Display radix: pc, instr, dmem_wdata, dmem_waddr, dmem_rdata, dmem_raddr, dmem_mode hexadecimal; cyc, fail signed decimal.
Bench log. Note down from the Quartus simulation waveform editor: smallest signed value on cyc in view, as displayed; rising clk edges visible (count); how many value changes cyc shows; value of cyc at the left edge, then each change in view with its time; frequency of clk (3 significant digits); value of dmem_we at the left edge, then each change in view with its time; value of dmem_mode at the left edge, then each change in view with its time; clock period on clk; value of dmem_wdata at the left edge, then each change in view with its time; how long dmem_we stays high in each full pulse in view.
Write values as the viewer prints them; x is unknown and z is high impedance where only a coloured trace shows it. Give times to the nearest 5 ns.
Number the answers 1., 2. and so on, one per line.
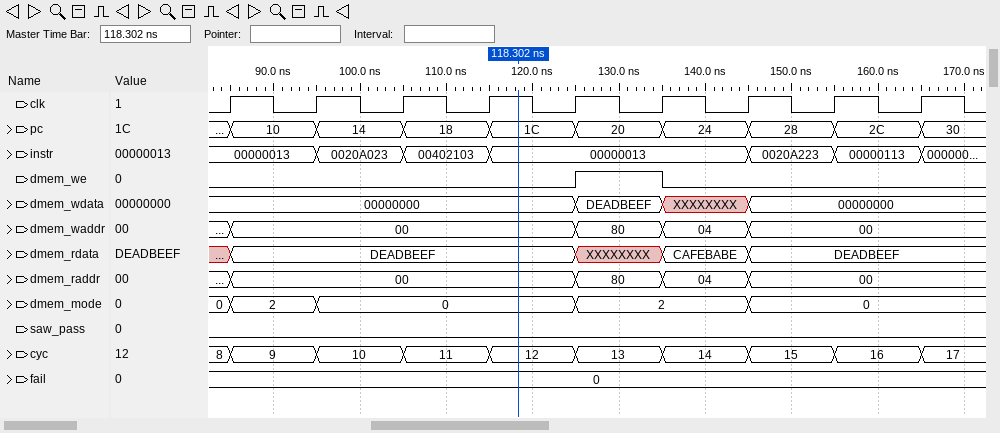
1. 8
2. 9
3. 9
4. 8, 9 at 85 ns, 10 at 95 ns, 11 at 105 ns, 12 at 115 ns, 13 at 125 ns, 14 at 135 ns, 15 at 145 ns, 16 at 155 ns, 17 at 165 ns
5. 100 MHz
6. 0, 1 at 125 ns, 0 at 135 ns
7. 0, 2 at 85 ns, 0 at 95 ns, 2 at 125 ns, 0 at 145 ns
8. 10 ns
9. 00000000, DEADBEEF at 125 ns, XXXXXXXX at 135 ns, 00000000 at 145 ns
10. 10 ns
